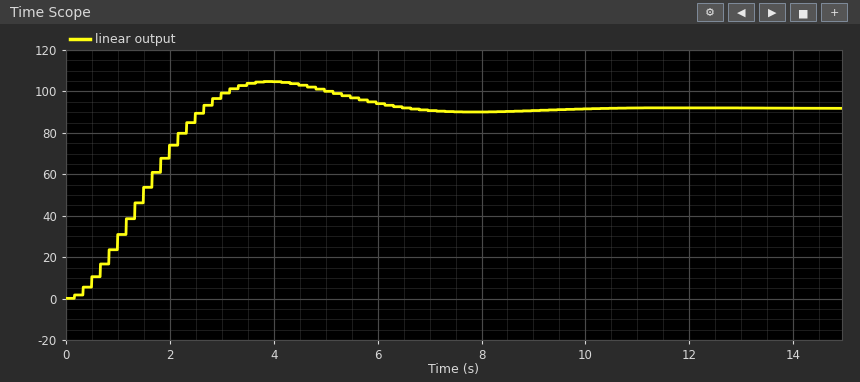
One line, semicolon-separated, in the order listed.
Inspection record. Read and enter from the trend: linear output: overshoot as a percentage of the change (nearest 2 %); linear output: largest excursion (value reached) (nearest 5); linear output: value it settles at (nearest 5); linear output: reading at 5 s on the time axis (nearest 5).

14 %; 105; 90; 100
